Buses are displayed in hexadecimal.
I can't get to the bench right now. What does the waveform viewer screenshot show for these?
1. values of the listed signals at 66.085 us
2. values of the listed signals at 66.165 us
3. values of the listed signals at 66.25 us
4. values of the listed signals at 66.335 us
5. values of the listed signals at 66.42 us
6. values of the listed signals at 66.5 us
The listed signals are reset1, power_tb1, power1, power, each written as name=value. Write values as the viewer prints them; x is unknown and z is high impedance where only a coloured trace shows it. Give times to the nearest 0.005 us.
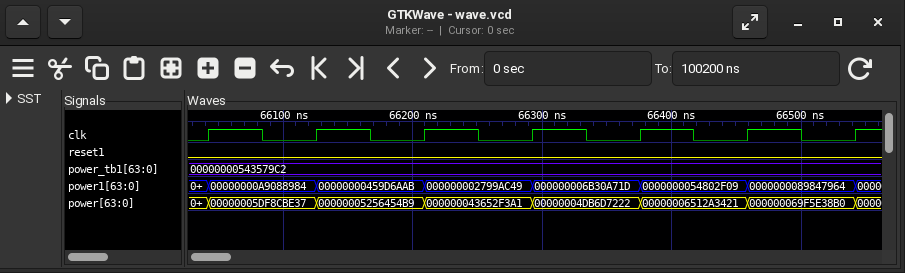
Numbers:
reset1=0, power_tb1=00000000543579C2, power1=00000000A9088984, power=00000005DF8CBE37
reset1=0, power_tb1=00000000543579C2, power1=00000000459D6AAB, power=00000005256454B9
reset1=0, power_tb1=00000000543579C2, power1=000000002799AC49, power=000000043652F3A1
reset1=0, power_tb1=00000000543579C2, power1=000000006B30A71D, power=00000004DB6D7222
reset1=0, power_tb1=00000000543579C2, power1=0000000054802F09, power=00000006512A3421
reset1=0, power_tb1=00000000543579C2, power1=0000000089847964, power=000000069F5E38B0
